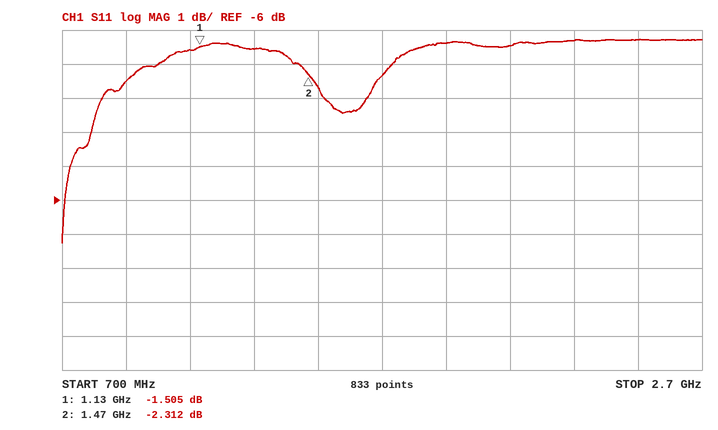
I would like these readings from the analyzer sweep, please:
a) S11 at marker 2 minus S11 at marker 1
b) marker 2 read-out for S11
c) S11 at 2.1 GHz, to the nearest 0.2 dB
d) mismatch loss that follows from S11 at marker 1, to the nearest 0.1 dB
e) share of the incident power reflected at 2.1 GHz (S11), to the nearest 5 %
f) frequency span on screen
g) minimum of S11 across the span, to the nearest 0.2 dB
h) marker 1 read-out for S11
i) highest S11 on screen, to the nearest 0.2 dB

-0.807 dB
-2.312 dB
-1.4 dB
5.3 dB
70 %
2 GHz
-7.2 dB
-1.505 dB
-1.2 dB
